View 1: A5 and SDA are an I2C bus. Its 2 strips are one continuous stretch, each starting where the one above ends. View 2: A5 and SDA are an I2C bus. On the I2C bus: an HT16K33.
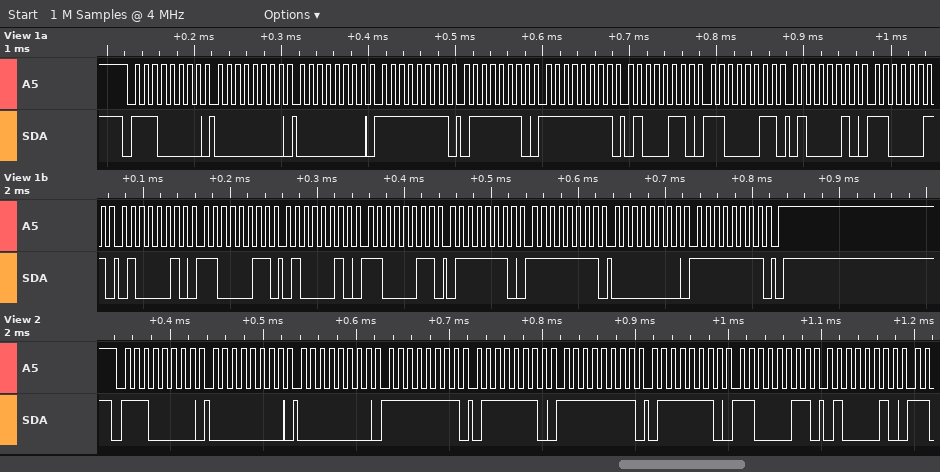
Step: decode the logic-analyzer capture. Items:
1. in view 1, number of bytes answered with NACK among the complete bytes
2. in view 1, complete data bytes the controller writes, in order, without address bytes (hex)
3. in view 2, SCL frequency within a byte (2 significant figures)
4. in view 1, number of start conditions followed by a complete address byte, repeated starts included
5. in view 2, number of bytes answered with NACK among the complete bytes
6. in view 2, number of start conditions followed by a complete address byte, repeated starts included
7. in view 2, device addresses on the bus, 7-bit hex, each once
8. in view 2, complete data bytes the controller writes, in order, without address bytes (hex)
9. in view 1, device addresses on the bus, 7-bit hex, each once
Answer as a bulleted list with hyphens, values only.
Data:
- 0
- 00 00 FF 7E FF 46 C3 42 C3 42 C3 42 C3 7E FF 00 FF
- 100 kHz
- 1
- 0
- 1
- 0x70
- 00 00 FF 7E FF 7E C3 42
- 0x70
